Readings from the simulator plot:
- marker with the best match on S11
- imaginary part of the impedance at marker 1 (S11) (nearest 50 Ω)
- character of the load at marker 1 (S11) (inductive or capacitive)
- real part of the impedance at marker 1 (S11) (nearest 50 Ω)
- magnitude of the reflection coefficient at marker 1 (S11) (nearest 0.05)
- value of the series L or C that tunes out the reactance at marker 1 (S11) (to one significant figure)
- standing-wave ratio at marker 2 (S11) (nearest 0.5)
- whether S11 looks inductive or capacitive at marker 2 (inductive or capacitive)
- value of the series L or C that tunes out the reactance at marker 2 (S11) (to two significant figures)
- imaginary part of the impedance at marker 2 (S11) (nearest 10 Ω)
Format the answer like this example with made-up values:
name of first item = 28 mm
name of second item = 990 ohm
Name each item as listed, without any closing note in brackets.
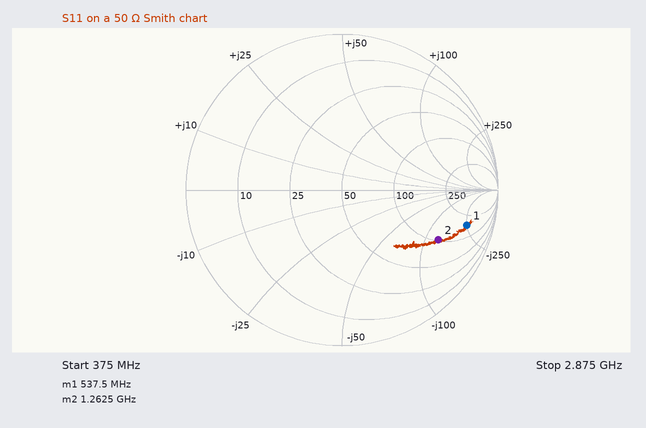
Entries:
marker with the best match on S11 = marker 2
imaginary part of the impedance at marker 1 (S11) = -250 Ω
character of the load at marker 1 (S11) = capacitive
real part of the impedance at marker 1 (S11) = 150 Ω
magnitude of the reflection coefficient at marker 1 (S11) = 0.85
value of the series L or C that tunes out the reactance at marker 1 (S11) = 70 nH
standing-wave ratio at marker 2 (S11) = 5.5
whether S11 looks inductive or capacitive at marker 2 = capacitive
value of the series L or C that tunes out the reactance at marker 2 (S11) = 16 nH
imaginary part of the impedance at marker 2 (S11) = -130 Ω
